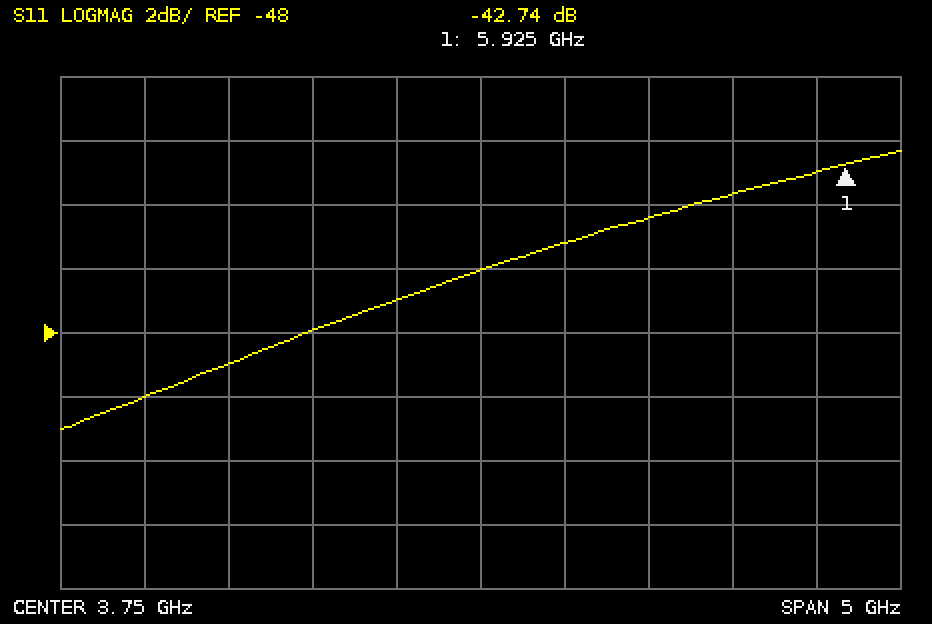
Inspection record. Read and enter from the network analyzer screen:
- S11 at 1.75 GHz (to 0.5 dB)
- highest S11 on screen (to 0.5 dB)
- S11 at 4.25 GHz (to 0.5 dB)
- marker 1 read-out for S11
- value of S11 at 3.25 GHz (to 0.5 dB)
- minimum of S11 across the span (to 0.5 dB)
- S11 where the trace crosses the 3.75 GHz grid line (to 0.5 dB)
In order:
-50.0 dB
-42.5 dB
-45.0 dB
-42.74 dB
-47.0 dB
-51.0 dB
-46.0 dB
